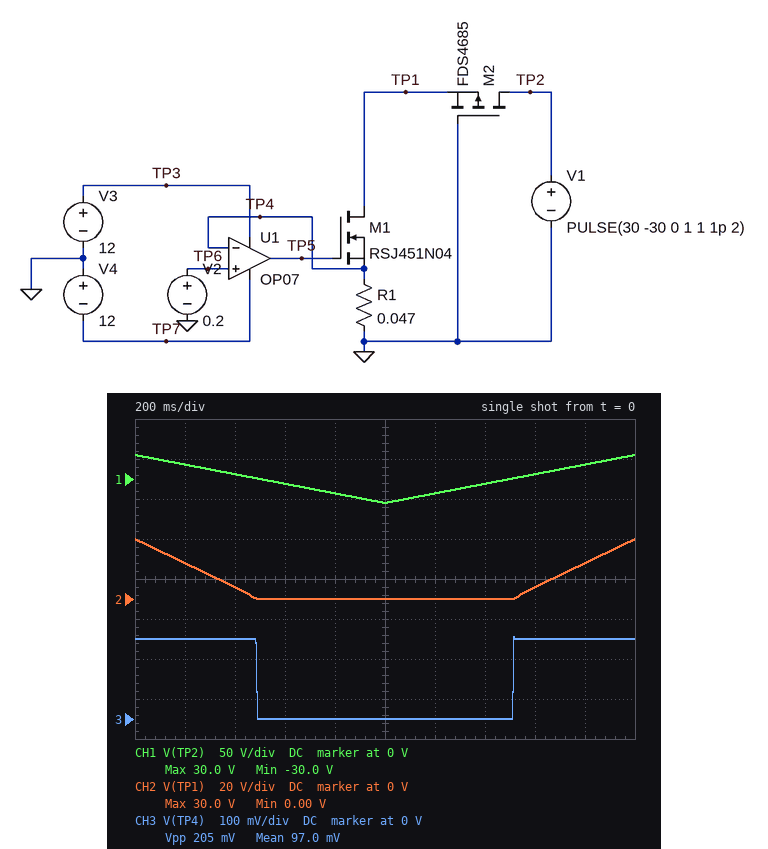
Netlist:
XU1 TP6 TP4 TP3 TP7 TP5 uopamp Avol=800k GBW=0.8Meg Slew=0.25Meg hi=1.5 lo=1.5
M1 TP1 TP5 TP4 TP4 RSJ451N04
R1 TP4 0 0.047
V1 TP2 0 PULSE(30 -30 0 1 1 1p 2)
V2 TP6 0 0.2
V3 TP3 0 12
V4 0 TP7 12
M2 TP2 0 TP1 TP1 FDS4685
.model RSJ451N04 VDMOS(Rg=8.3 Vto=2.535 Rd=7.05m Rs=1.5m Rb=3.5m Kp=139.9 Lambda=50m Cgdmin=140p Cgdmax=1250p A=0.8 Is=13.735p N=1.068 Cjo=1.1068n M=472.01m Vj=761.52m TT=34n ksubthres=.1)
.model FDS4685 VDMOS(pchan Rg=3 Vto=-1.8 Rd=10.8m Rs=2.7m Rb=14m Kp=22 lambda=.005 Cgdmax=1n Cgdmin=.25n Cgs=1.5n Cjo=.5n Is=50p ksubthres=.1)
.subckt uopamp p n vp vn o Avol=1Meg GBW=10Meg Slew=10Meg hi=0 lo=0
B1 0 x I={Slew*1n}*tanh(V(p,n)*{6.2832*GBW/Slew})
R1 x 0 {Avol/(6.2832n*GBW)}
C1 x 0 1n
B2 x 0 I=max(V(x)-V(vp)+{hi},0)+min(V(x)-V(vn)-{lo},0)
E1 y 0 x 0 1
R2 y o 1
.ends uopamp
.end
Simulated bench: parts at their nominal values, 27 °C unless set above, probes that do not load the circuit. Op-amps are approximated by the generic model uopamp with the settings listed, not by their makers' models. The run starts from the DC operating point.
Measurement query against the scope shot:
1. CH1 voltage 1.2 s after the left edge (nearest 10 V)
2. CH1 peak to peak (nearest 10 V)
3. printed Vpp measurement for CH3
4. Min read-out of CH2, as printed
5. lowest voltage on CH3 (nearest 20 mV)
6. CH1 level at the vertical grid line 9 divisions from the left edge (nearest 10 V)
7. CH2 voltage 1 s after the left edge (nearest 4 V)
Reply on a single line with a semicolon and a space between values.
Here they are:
-20 V; 60 V; 205 mV; 0.00 V; 0 V; 20 V; 0 V
